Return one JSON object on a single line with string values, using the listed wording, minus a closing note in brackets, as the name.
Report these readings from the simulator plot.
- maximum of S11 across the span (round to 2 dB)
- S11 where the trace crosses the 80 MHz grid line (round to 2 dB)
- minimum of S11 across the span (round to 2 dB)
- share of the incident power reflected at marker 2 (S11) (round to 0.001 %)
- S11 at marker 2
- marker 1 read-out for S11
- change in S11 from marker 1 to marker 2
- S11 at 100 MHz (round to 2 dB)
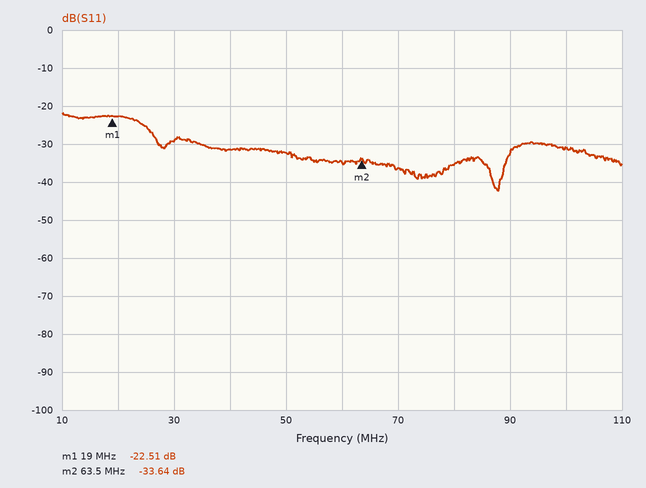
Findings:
{"maximum of S11 across the span": "-22 dB", "S11 where the trace crosses the 80 MHz grid line": "-36 dB", "minimum of S11 across the span": "-42 dB", "share of the incident power reflected at marker 2 (S11)": "0.043 %", "S11 at marker 2": "-33.64 dB", "marker 1 read-out for S11": "-22.51 dB", "change in S11 from marker 1 to marker 2": "-11.13 dB", "S11 at 100 MHz": "-30 dB"}
